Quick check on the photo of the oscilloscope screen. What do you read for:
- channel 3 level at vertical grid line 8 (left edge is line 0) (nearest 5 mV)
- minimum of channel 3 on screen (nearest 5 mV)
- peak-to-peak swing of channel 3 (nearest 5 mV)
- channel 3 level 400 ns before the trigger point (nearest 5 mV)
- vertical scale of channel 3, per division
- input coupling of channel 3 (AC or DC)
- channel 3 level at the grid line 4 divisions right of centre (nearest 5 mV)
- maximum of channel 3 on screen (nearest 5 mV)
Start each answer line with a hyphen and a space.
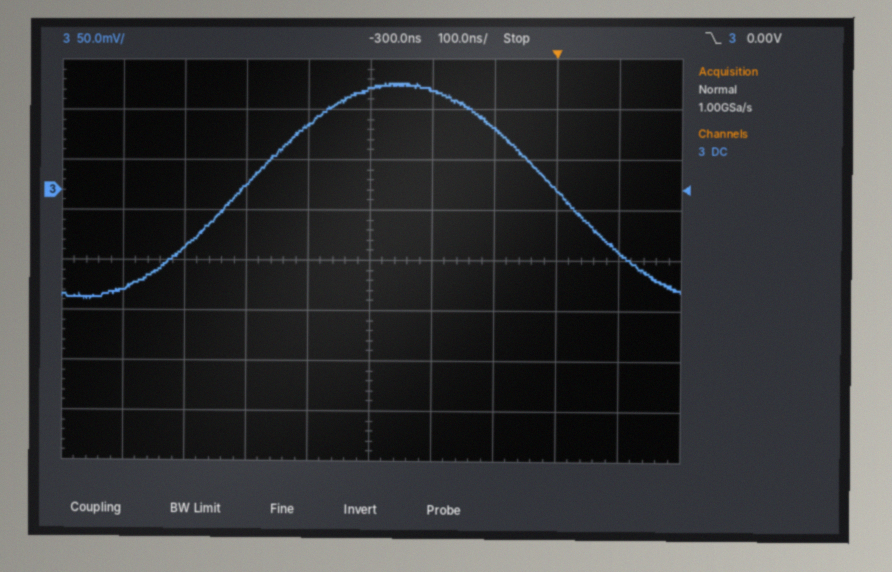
- 0 mV
- -110 mV
- 215 mV
- 65 mV
- 50 mV
- DC
- -60 mV
- 105 mV
